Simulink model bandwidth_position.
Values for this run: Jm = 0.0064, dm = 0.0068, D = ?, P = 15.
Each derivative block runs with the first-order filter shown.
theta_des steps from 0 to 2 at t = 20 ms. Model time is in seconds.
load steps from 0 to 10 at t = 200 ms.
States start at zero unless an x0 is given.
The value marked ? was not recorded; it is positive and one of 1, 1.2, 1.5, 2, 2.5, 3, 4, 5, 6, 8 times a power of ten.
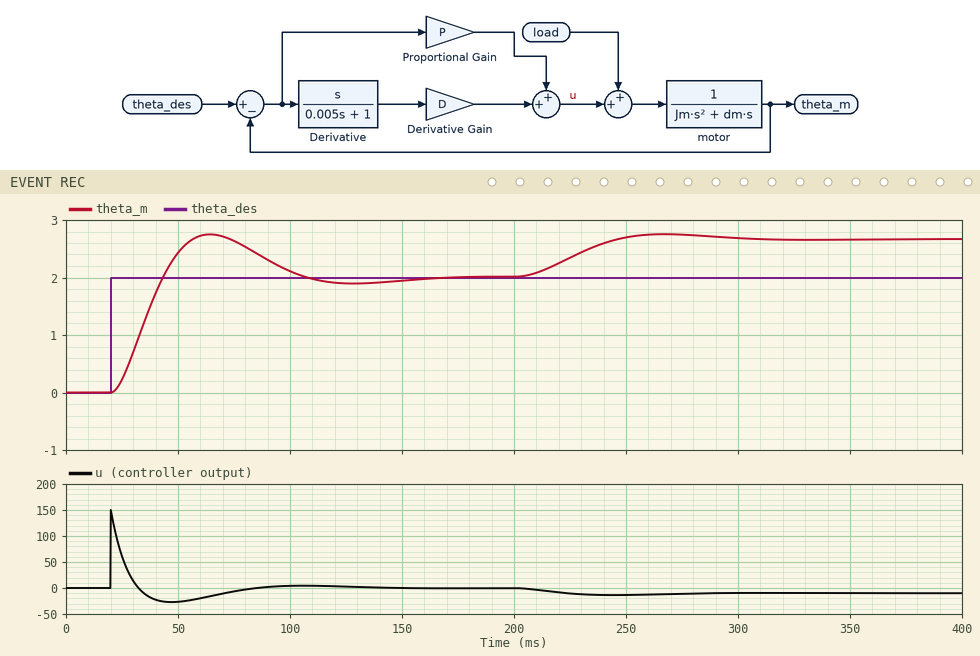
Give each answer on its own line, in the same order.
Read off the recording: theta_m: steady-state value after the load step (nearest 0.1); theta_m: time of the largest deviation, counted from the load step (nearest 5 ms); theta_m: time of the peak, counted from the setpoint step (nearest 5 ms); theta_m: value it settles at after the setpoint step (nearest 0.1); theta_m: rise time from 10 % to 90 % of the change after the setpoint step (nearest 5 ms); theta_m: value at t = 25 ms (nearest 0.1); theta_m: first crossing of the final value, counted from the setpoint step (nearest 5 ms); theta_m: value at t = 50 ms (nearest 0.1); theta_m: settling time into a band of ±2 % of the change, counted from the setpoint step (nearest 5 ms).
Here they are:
2.7
65 ms
45 ms
2.0
15 ms
0.2
25 ms
2.4
135 ms
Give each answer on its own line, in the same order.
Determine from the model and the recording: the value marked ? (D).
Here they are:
0.3
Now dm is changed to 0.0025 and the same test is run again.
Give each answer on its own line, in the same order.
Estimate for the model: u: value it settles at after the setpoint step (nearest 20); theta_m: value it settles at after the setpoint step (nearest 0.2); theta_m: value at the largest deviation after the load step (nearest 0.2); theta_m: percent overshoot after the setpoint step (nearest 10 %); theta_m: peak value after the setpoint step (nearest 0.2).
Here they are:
0
2.0
2.8
40 %
2.8
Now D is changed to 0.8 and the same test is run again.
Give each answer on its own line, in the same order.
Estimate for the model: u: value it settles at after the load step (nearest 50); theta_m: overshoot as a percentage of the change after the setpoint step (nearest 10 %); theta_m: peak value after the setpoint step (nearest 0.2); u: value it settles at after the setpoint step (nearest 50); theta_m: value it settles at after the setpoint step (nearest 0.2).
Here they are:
0
20 %
2.4
0
2.0
